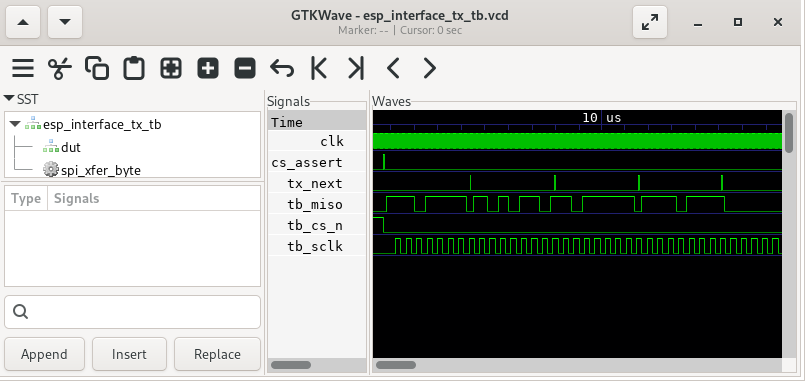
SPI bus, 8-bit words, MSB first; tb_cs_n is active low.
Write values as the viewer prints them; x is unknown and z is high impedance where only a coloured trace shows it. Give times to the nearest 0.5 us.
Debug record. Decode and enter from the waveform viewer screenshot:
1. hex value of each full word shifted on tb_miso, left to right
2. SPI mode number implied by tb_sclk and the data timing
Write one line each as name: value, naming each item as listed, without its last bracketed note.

hex value of each full word shifted on tb_miso, left to right: DE, AD, BE, EF
SPI mode number implied by tb_sclk and the data timing: 0
